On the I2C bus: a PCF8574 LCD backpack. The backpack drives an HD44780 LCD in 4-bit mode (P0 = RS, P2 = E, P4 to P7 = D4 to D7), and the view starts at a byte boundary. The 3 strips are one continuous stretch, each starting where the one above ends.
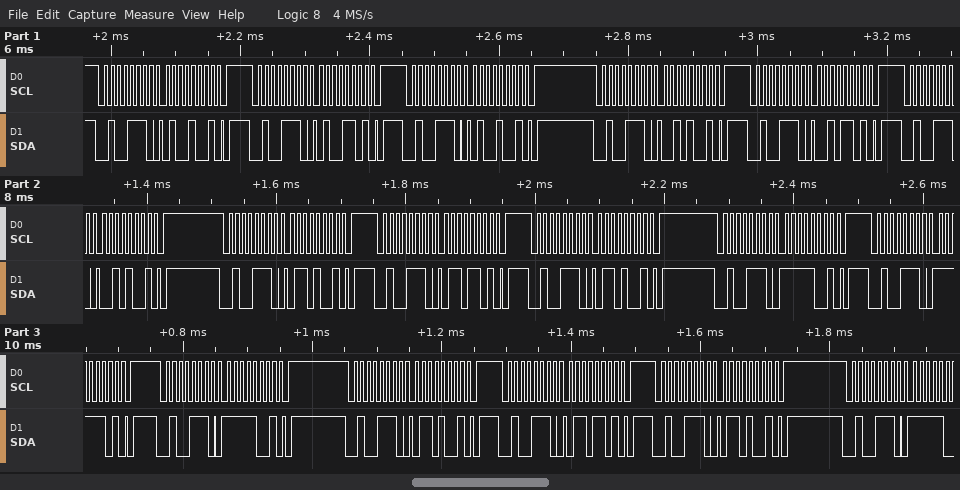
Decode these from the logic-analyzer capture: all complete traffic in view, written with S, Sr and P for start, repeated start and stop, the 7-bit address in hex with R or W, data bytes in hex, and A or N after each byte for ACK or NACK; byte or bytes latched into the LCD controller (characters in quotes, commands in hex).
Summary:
S 27W A 49 A P S 27W A 4D A P S 27W A 49 A P S 27W A 29 A P S 27W A 2D A P S 27W A 29 A P S 27W A 69 A P S 27W A 6D A P S 27W A 69 A P S 27W A F9 A P S 27W A FD A P S 27W A F9 A P S 27W A 69 A P S 27W A 6D A P S 27W A 69 A P S 27W A
'B' 'o'
